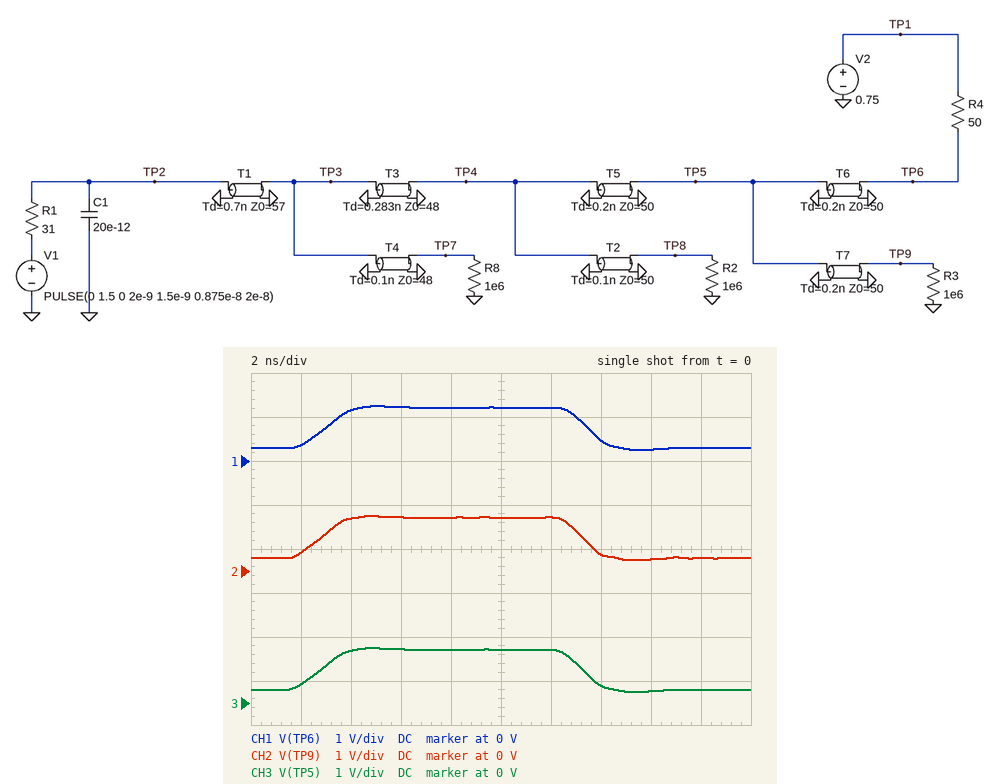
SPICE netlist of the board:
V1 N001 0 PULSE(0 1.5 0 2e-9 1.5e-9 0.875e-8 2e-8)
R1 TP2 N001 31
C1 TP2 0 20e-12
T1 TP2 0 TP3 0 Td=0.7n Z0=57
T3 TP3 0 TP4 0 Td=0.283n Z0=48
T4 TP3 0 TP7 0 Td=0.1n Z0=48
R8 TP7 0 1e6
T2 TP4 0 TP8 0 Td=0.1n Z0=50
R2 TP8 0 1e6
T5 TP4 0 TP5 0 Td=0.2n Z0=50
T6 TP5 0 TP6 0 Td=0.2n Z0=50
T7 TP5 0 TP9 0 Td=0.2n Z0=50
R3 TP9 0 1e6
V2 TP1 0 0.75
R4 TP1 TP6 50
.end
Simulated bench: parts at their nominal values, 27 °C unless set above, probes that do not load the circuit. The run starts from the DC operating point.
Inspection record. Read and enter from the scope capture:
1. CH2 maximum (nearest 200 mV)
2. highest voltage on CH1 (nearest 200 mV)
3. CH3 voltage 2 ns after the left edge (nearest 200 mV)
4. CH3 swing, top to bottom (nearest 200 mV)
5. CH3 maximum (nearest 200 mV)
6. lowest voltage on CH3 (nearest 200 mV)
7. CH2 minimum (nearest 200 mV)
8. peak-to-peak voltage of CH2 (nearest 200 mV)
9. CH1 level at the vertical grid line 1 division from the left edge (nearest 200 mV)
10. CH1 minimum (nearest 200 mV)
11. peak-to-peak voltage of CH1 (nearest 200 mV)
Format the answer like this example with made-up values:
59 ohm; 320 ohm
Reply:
1.2 V; 1.2 V; 400 mV; 1.0 V; 1.2 V; 200 mV; 200 mV; 1.0 V; 400 mV; 200 mV; 1.0 V
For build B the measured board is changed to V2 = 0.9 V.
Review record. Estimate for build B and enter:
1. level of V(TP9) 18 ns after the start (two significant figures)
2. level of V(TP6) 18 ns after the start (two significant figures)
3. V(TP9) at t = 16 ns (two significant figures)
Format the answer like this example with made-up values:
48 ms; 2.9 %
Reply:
360 mV; 350 mV; 320 mV
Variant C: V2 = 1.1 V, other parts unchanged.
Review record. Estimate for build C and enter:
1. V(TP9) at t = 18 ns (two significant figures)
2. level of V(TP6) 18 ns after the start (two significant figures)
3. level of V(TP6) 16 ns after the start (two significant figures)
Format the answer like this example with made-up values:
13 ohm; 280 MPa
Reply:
440 mV; 430 mV; 390 mV
